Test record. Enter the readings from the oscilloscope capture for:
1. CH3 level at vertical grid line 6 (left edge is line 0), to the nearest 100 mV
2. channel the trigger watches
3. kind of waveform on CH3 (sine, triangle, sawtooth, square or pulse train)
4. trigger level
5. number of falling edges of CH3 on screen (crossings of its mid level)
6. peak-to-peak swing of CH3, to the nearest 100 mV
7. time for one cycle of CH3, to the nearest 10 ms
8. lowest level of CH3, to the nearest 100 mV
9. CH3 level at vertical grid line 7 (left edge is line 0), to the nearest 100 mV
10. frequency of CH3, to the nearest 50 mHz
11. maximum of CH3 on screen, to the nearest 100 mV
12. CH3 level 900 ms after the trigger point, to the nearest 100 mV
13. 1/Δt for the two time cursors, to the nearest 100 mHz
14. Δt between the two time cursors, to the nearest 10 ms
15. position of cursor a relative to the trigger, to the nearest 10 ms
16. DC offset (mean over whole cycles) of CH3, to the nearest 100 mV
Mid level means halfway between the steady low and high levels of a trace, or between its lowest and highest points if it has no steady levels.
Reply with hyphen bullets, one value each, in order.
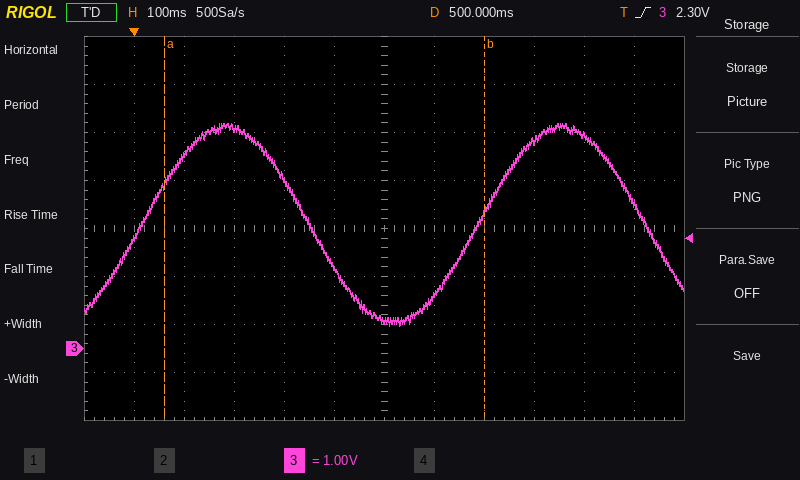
- 600 mV
- CH3
- sine
- 2.30 V
- 2
- 4.2 V
- 670 ms
- 500 mV
- 1.1 V
- 1.50 Hz
- 4.7 V
- 4.4 V
- 1.6 Hz
- 640 ms
- +60 ms
- 2.6 V
